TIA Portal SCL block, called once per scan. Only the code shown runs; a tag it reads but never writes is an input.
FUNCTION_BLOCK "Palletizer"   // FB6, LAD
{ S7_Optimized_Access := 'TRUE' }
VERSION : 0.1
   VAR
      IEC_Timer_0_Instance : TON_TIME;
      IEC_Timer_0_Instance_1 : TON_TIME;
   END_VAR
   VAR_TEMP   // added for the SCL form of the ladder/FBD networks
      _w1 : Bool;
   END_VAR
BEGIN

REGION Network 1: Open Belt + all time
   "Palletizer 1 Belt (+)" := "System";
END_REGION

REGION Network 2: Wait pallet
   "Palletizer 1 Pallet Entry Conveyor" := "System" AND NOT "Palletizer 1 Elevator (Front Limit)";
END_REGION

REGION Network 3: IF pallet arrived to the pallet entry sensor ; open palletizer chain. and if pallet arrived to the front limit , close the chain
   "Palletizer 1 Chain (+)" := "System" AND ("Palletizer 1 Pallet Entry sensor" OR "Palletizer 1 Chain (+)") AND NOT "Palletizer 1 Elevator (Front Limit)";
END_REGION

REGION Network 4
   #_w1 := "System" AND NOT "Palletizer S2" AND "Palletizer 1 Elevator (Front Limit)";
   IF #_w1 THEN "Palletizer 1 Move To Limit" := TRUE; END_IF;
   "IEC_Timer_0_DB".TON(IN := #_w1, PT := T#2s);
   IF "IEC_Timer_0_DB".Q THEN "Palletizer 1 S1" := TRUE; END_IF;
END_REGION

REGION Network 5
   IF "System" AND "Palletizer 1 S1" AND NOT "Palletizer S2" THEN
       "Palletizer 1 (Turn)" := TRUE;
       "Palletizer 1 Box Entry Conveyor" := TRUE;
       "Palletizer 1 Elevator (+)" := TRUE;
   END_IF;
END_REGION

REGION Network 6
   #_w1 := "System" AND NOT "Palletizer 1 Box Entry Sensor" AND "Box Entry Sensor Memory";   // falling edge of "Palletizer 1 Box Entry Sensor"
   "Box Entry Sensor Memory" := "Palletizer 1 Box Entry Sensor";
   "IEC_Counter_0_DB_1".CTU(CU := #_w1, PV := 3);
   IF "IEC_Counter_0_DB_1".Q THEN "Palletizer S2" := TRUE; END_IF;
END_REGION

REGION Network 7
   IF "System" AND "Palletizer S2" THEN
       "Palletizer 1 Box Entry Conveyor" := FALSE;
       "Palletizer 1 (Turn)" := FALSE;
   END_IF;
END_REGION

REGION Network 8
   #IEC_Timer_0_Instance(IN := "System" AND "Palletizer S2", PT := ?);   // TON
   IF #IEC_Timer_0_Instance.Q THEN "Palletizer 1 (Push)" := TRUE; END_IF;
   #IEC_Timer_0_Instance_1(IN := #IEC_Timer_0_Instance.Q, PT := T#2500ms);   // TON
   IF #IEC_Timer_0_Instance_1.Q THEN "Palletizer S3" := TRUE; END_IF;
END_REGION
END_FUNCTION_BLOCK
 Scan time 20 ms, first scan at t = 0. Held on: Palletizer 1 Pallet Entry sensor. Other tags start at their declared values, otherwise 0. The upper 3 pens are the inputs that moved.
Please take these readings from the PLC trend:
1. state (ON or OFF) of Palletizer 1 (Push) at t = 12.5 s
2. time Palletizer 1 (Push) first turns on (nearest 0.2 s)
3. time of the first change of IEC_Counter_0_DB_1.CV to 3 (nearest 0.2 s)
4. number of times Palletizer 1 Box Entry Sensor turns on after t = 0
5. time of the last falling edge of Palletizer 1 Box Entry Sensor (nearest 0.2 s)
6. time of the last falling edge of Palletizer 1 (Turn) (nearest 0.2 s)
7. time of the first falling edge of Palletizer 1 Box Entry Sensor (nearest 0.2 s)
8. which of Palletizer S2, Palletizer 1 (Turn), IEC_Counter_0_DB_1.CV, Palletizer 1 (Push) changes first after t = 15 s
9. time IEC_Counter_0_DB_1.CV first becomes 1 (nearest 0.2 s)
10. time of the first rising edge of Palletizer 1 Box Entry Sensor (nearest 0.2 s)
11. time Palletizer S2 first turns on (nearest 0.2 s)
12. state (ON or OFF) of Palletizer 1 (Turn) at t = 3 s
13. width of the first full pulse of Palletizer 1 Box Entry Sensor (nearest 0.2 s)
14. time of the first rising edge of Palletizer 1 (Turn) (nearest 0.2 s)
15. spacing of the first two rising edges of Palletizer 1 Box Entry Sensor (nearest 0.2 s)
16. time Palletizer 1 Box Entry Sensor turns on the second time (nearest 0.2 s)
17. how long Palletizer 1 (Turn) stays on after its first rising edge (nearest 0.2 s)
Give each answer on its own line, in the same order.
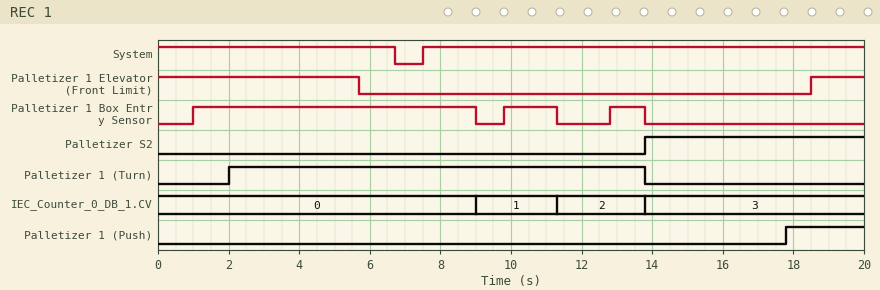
OFF
17.8 s
13.8 s
3
13.8 s
13.8 s
9.0 s
Palletizer 1 (Push)
9.0 s
1.0 s
13.8 s
ON
8.0 s
2.0 s
8.8 s
9.8 s
11.8 s
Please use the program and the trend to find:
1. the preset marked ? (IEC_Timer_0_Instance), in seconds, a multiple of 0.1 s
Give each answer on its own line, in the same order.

4.0 s
